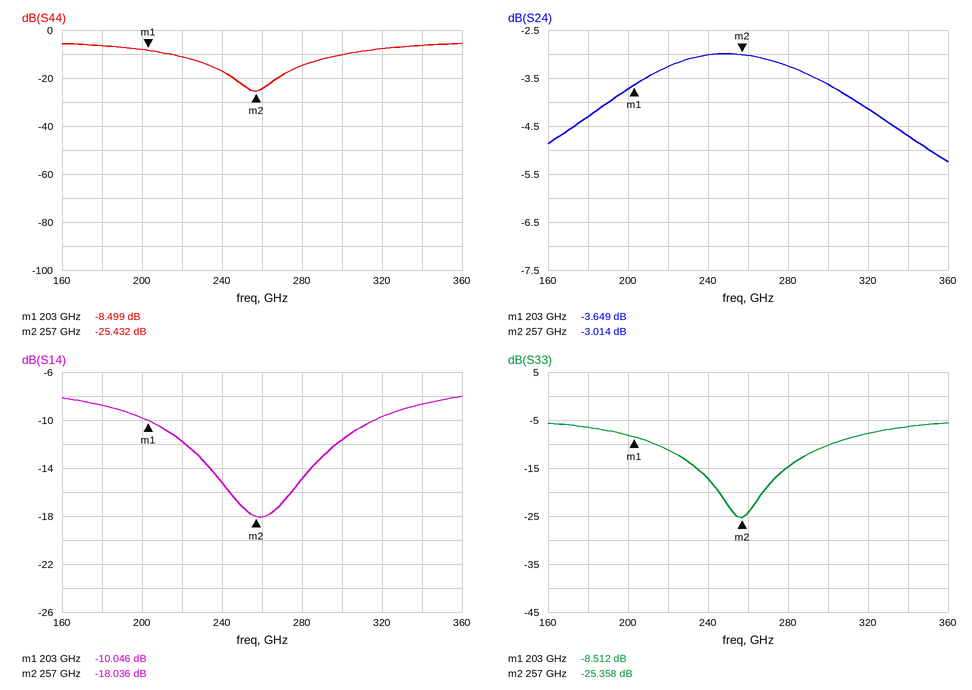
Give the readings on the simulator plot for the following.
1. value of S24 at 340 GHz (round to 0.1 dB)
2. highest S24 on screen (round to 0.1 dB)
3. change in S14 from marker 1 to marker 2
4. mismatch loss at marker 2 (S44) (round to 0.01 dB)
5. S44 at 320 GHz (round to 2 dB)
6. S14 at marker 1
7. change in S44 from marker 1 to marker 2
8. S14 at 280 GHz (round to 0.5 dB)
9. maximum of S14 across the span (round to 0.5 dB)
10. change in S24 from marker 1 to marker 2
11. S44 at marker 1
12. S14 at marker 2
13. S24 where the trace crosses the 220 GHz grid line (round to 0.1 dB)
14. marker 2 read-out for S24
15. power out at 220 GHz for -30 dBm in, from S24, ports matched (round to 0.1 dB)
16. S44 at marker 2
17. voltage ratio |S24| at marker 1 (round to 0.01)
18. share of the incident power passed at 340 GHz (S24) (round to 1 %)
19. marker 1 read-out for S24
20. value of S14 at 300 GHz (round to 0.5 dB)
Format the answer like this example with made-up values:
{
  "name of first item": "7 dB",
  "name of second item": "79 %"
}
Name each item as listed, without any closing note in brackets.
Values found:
{
  "value of S24 at 340 GHz": "-4.7 dB",
  "highest S24 on screen": "-3.0 dB",
  "change in S14 from marker 1 to marker 2": "-7.990 dB",
  "mismatch loss at marker 2 (S44)": "0.01 dB",
  "S44 at 320 GHz": "-8 dB",
  "S14 at marker 1": "-10.046 dB",
  "change in S44 from marker 1 to marker 2": "-16.933 dB",
  "S14 at 280 GHz": "-15.0 dB",
  "maximum of S14 across the span": "-8.0 dB",
  "change in S24 from marker 1 to marker 2": "0.635 dB",
  "S44 at marker 1": "-8.499 dB",
  "S14 at marker 2": "-18.036 dB",
  "S24 where the trace crosses the 220 GHz grid line": "-3.3 dB",
  "marker 2 read-out for S24": "-3.014 dB",
  "power out at 220 GHz for -30 dBm in, from S24, ports matched": "-33.3 dBm",
  "S44 at marker 2": "-25.432 dB",
  "voltage ratio |S24| at marker 1": "0.66",
  "share of the incident power passed at 340 GHz (S24)": "34 %",
  "marker 1 read-out for S24": "-3.649 dB",
  "value of S14 at 300 GHz": "-11.5 dB"
}
